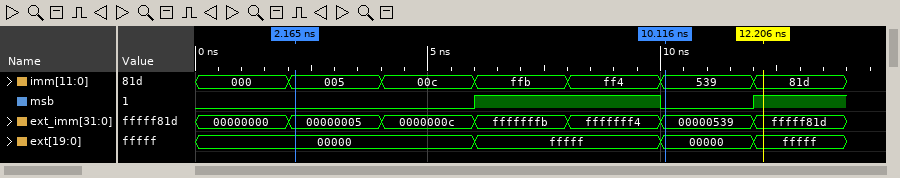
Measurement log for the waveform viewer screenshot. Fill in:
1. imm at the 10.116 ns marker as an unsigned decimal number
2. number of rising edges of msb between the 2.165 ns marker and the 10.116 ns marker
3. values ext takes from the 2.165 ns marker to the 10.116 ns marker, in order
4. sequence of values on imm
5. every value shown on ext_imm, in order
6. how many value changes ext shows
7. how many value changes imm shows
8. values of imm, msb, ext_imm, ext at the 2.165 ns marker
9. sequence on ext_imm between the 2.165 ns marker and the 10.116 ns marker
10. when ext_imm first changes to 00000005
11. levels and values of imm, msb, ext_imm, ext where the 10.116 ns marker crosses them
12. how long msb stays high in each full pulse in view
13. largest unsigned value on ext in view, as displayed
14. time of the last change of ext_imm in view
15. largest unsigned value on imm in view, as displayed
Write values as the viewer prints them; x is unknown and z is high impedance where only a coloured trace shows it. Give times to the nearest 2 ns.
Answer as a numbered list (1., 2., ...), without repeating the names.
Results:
1. 1337
2. 1
3. 00000, fffff, 00000
4. 000, 005, 00c, ffb, ff4, 539, 81d
5. 00000000, 00000005, 0000000c, fffffffb, fffffff4, 00000539, fffff81d
6. 3
7. 6
8. imm=005, msb=0, ext_imm=00000005, ext=00000
9. 00000005, 0000000c, fffffffb, fffffff4, 00000539
10. 2 ns
11. imm=539, msb=0, ext_imm=00000539, ext=00000
12. 4 ns
13. fffff
14. 12 ns
15. ffb
